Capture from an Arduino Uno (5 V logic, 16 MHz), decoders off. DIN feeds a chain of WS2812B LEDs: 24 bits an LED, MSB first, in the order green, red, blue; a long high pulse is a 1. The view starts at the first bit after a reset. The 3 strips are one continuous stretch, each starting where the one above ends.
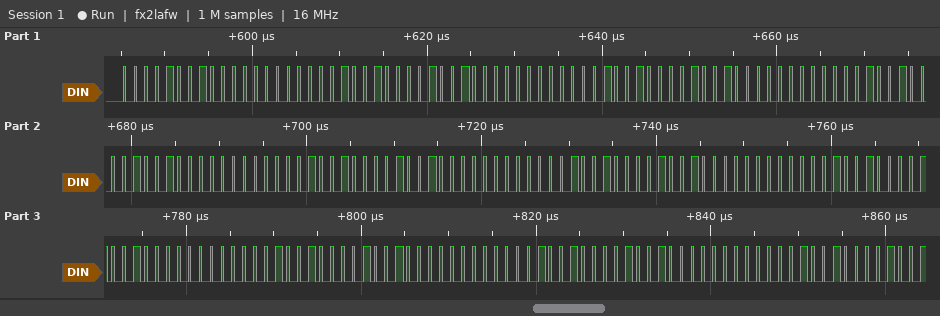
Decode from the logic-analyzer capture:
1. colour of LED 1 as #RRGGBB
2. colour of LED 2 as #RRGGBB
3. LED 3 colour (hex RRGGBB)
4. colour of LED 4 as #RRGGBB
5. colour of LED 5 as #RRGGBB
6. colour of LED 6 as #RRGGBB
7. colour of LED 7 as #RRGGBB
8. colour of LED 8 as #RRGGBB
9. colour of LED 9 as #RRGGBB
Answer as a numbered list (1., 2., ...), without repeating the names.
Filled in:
1. #000909
2. #000909
3. #000909
4. #000909
5. #000909
6. #000909
7. #000909
8. #000909
9. #000909
